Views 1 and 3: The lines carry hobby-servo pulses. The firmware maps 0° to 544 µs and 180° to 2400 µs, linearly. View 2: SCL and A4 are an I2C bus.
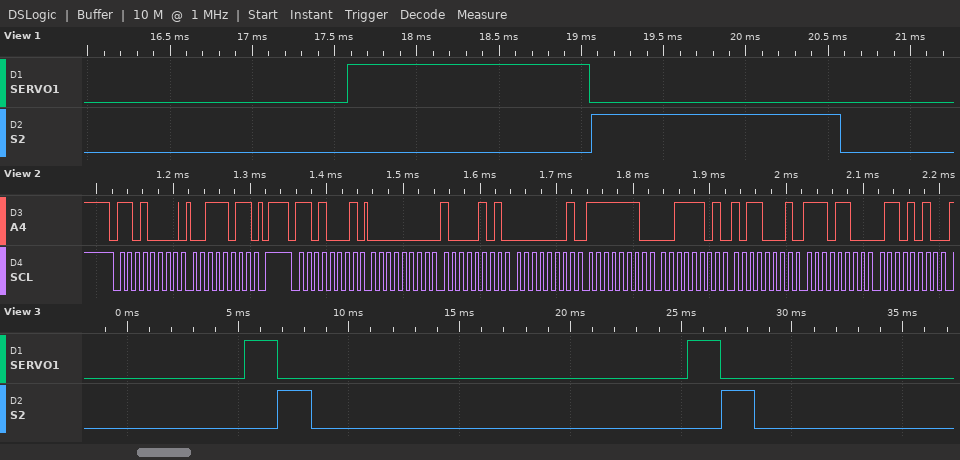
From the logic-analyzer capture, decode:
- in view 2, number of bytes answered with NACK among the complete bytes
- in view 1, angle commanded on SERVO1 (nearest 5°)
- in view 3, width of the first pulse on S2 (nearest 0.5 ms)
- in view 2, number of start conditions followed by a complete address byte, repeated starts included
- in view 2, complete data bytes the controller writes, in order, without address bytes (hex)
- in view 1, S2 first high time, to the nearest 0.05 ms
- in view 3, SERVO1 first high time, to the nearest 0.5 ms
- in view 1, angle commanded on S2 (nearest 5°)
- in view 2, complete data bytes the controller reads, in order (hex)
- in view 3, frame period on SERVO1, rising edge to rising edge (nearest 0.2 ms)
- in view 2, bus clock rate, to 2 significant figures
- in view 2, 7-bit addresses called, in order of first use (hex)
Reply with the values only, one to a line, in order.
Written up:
0
90°
1.5 ms
2
3B
1.50 ms
1.5 ms
95°
00 85 01 FE 3D B1 EC 6A
20.0 ms
100 kHz
0x68
